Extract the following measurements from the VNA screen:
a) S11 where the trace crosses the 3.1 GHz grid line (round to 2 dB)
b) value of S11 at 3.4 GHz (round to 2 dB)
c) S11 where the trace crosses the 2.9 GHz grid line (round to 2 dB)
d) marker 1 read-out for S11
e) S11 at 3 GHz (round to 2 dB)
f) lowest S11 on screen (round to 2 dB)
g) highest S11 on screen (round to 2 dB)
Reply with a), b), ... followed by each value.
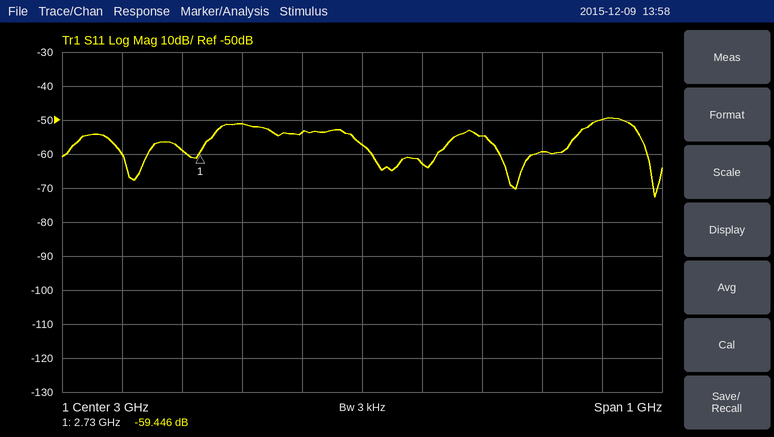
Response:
a) -62 dB
b) -50 dB
c) -54 dB
d) -59.446 dB
e) -58 dB
f) -72 dB
g) -50 dB
